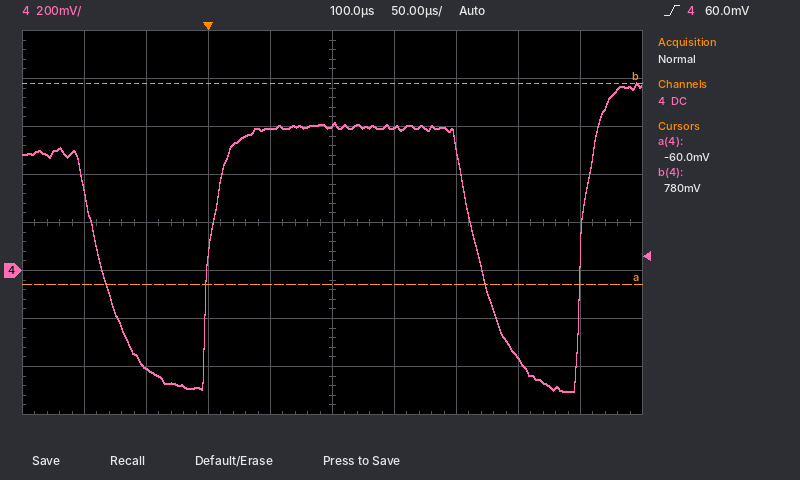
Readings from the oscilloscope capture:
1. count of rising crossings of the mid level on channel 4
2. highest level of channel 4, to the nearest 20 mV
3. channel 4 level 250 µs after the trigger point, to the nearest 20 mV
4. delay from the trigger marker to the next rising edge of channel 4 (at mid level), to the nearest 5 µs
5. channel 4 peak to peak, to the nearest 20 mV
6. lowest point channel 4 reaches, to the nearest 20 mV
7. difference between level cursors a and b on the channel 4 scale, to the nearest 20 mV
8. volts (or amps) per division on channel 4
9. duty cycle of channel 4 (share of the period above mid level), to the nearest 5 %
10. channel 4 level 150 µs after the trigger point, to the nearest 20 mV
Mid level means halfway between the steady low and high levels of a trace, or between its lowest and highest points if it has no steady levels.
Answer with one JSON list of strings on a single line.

["2", "780 mV", "-360 mV", "300 µs", "1.28 V", "-500 mV", "840 mV", "200 mV", "70 %", "600 mV"]
